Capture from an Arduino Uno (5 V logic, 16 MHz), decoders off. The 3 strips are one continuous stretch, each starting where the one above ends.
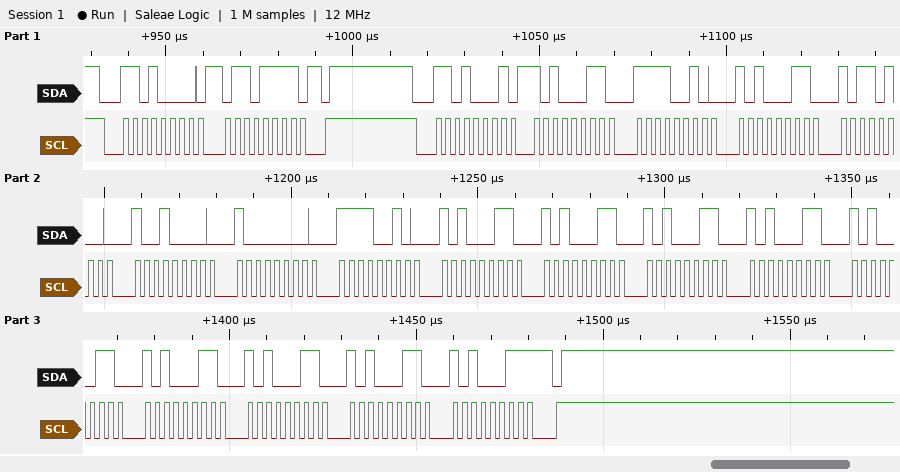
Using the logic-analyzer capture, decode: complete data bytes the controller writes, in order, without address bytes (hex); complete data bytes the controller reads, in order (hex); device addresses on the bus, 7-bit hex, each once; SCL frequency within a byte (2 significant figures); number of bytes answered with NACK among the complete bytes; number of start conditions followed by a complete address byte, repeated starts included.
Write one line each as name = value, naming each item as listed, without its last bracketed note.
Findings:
complete data bytes the controller writes, in order, without address bytes = 6F
complete data bytes the controller reads, in order = A3 F2 A3 B4 90 80 F2 A3 A3 A3 A3 A3 A3 A3 A3 A3
device addresses on the bus, 7-bit hex, each once = 0x68
SCL frequency within a byte = 400 kHz
number of bytes answered with NACK among the complete bytes = 1
number of start conditions followed by a complete address byte, repeated starts included = 2
